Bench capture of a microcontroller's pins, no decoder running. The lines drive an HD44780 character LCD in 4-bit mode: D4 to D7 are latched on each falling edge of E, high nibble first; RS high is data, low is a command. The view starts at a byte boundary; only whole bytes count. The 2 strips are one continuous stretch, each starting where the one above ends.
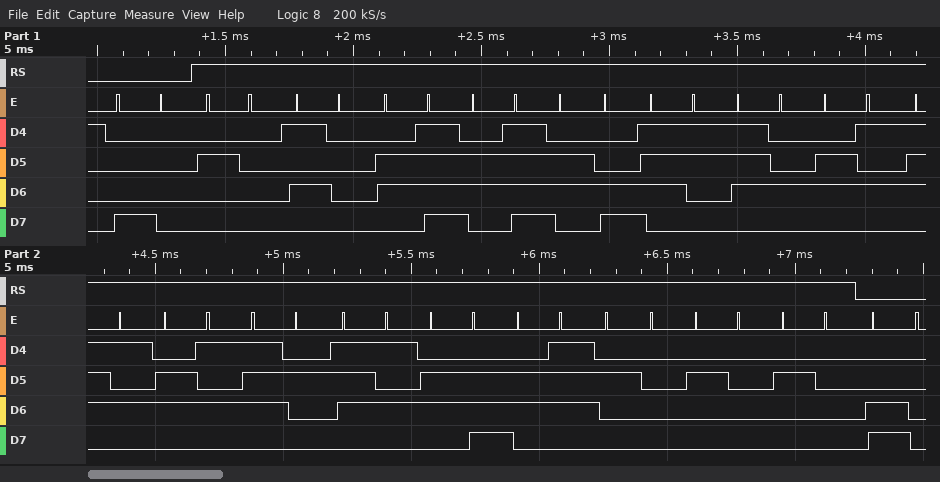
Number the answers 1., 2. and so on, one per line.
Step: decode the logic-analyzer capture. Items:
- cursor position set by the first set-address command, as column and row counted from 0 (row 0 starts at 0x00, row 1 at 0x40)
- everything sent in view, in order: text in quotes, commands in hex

1. column 0, row 0
2. 0x80 " Poolsteuerung   " 0xC0
